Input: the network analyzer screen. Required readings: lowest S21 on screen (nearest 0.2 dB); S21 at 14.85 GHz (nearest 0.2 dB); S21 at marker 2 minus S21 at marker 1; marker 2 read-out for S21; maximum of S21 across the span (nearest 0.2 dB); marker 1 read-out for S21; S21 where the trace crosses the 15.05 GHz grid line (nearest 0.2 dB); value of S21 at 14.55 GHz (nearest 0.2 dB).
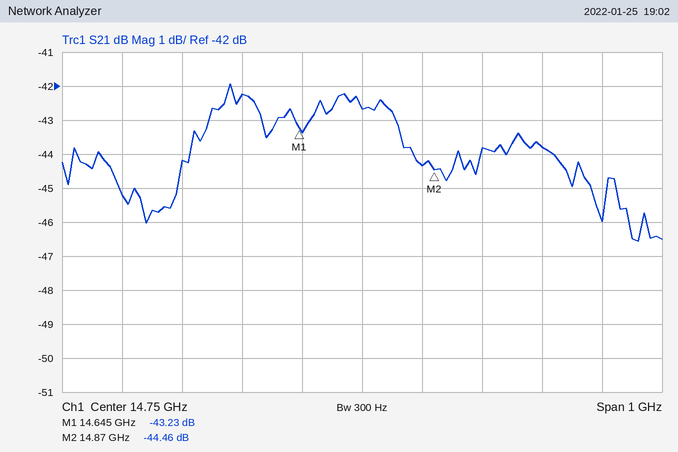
-46.6 dB
-44.4 dB
-1.23 dB
-44.46 dB
-42.0 dB
-43.23 dB
-43.8 dB
-42.2 dB
